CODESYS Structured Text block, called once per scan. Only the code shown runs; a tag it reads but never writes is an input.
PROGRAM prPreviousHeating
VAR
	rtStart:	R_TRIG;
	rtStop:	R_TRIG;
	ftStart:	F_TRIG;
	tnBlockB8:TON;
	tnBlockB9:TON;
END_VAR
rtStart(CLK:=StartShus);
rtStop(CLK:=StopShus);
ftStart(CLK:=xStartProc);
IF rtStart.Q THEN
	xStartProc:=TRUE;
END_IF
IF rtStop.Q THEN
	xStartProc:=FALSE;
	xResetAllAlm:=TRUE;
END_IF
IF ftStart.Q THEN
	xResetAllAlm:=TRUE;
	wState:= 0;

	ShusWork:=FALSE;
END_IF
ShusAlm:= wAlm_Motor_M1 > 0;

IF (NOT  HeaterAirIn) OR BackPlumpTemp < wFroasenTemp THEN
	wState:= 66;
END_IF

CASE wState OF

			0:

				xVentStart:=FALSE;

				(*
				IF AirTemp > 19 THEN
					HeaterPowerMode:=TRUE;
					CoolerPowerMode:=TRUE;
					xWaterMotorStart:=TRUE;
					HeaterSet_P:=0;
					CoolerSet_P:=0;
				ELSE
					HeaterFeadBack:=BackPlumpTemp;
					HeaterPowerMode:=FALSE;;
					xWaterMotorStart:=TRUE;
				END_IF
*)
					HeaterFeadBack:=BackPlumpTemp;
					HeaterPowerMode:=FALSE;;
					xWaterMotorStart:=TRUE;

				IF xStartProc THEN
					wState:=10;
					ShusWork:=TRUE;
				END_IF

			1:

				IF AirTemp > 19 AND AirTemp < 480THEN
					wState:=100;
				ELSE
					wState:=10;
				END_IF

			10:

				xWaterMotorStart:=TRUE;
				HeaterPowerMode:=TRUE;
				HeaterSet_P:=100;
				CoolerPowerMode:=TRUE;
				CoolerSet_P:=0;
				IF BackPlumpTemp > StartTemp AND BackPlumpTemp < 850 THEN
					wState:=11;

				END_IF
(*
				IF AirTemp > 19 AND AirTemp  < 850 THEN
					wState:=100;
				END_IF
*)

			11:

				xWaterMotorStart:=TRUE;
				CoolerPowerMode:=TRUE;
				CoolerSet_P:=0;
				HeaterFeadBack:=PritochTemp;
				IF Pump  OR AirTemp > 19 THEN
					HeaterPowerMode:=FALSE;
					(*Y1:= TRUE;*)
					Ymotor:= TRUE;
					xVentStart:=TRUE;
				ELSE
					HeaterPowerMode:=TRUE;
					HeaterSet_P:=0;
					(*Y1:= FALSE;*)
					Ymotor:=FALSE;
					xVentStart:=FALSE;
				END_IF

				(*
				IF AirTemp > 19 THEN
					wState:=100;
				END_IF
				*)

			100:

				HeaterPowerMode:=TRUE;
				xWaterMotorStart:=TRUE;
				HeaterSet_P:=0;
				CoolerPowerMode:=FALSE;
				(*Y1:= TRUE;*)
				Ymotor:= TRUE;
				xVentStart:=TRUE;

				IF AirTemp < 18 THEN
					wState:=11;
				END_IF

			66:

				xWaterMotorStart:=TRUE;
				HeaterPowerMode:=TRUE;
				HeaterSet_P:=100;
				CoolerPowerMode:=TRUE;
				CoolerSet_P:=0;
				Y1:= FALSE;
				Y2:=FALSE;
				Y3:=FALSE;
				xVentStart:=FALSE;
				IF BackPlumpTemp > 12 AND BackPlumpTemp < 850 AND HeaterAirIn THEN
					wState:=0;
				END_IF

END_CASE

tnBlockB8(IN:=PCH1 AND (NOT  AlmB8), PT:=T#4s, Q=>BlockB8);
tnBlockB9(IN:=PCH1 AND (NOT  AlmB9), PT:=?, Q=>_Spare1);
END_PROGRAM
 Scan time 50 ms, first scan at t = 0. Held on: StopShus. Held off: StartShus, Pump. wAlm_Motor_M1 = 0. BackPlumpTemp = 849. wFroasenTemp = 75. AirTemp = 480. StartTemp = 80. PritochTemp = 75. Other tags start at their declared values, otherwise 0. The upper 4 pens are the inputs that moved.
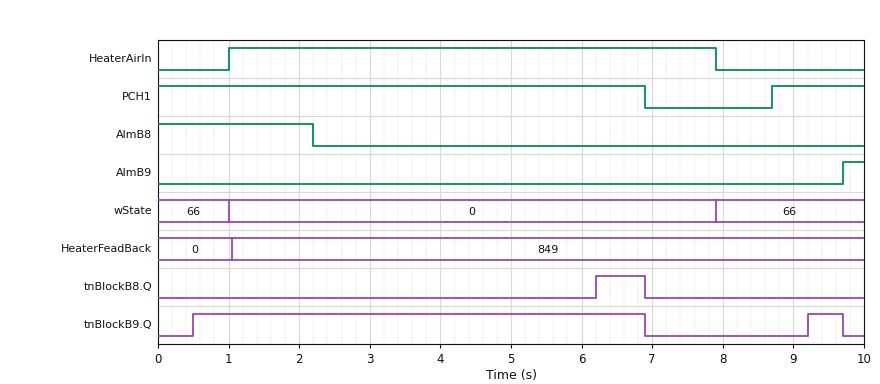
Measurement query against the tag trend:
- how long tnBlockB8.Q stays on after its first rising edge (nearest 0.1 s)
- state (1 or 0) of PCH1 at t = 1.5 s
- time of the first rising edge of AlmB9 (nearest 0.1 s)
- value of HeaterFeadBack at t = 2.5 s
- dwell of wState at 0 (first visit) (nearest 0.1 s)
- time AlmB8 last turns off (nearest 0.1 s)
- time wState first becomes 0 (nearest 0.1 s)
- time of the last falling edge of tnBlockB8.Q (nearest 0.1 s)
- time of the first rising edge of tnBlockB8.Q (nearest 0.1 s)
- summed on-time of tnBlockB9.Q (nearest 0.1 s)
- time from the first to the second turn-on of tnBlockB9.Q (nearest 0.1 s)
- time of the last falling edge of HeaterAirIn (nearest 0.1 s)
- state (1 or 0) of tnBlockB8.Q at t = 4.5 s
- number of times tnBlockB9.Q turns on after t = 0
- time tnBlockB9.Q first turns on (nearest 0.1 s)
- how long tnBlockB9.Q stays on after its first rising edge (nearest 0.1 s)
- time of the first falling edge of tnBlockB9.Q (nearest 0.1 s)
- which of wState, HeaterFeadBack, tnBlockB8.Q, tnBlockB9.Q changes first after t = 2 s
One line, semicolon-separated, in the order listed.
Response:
0.7 s; 1; 9.7 s; 849; 6.9 s; 2.2 s; 1.0 s; 6.9 s; 6.2 s; 6.9 s; 8.7 s; 7.9 s; 0; 2; 0.5 s; 6.4 s; 6.9 s; tnBlockB8.Q
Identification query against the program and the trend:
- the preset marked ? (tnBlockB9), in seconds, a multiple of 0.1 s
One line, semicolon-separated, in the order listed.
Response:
0.5 s
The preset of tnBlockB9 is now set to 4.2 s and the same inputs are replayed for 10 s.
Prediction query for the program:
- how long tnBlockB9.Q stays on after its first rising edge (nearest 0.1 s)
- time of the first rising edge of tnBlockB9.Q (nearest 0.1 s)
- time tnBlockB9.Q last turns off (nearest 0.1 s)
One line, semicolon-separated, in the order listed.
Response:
2.7 s; 4.2 s; 6.9 s
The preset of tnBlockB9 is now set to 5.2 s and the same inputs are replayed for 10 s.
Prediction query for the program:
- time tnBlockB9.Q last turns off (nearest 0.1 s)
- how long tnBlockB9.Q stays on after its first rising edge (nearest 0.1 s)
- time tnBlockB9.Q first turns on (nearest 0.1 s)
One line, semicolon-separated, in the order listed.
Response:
6.9 s; 1.7 s; 5.2 s
